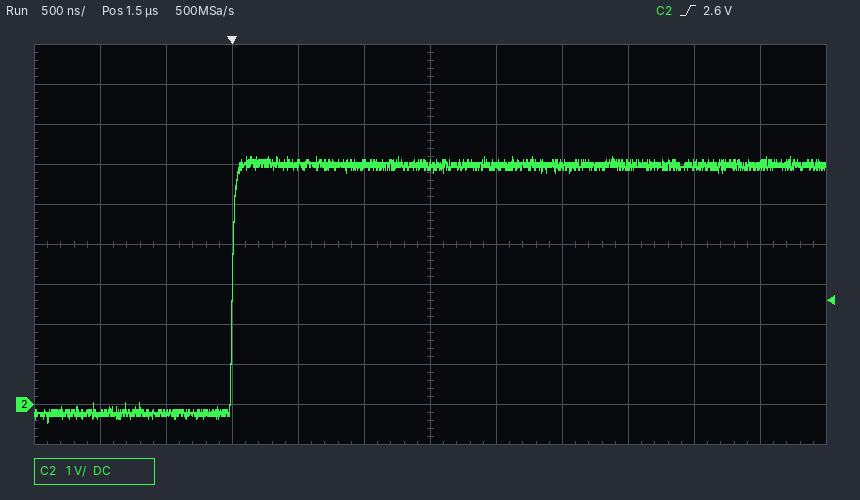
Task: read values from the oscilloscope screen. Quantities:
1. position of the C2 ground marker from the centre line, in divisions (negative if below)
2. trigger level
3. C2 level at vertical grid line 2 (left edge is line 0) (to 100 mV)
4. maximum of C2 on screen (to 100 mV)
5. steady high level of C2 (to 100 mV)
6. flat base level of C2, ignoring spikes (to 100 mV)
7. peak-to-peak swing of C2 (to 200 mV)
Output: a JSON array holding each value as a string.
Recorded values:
["-4.0 div", "2.6 V", "-200 mV", "6.2 V", "6.0 V", "-200 mV", "6.6 V"]
